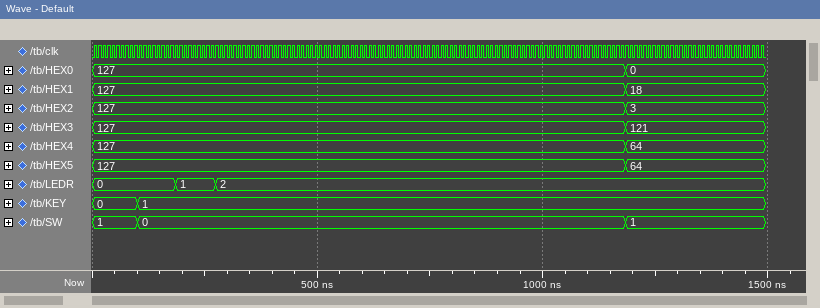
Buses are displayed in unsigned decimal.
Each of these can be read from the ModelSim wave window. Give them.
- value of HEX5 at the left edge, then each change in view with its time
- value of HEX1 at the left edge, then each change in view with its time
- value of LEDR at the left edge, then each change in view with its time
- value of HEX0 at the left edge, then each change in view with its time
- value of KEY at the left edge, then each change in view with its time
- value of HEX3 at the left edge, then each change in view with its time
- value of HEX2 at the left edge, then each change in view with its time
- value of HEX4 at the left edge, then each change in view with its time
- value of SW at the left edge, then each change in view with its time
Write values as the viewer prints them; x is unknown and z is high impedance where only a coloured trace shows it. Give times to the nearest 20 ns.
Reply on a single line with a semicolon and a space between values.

127, 64 at 1180 ns; 127, 18 at 1180 ns; 0, 1 at 180 ns, 2 at 280 ns; 127, 0 at 1180 ns; 0, 1 at 100 ns; 127, 121 at 1180 ns; 127, 3 at 1180 ns; 127, 64 at 1180 ns; 1, 0 at 100 ns, 1 at 1180 ns
